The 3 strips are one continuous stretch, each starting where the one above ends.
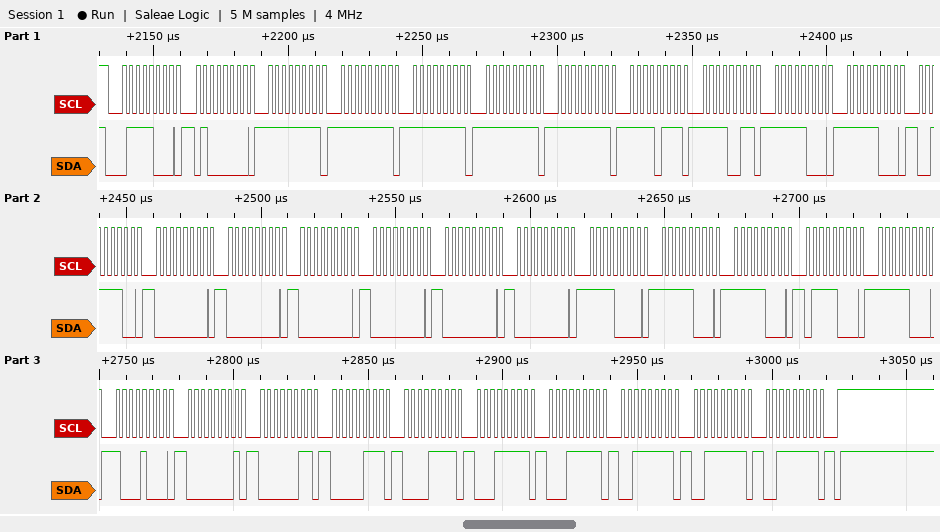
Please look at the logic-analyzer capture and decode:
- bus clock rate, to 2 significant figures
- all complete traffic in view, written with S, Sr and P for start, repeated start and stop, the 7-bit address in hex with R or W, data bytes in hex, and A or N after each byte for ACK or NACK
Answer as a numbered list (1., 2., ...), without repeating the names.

1. 400 kHz
2. S 3CW A 40 A FF A FF A FF A FF A FF A F7 A F3 A F8 A F8 A 3C A 00 A 00 A 00 A 00 A 00 A 00 A F0 A F8 A F8 A 78 A F8 A 88 A 01 A 03 A 07 A 0F A 1F A 1F A 3F A 3F A 3F A P
